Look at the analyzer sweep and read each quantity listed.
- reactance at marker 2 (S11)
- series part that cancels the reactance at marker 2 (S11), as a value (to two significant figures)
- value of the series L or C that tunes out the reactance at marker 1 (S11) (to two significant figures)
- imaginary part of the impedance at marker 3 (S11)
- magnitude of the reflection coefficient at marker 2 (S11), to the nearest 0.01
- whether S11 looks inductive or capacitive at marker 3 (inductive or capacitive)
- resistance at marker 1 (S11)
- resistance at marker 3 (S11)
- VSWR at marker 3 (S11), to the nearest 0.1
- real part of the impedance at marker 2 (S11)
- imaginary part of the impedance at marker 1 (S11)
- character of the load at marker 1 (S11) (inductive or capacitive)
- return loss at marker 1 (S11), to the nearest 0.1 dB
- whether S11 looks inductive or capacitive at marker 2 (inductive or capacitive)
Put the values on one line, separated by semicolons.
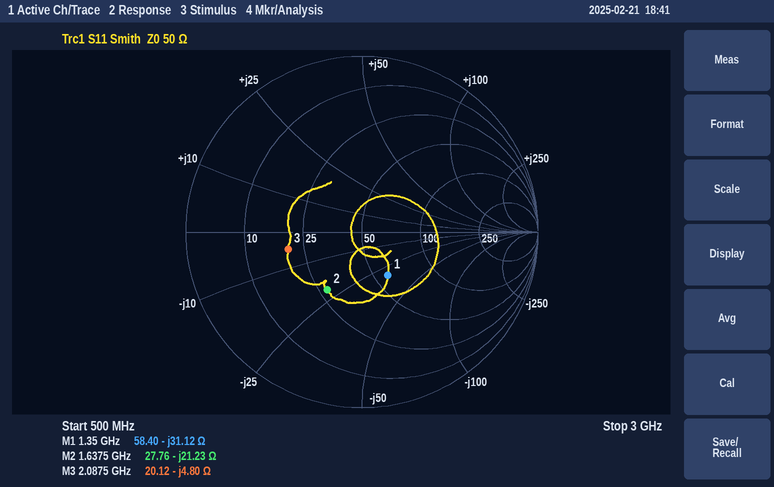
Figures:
-21.23 Ω; 2.1 nH; 3.7 nH; -4.80 Ω; 0.38; capacitive; 58.40 Ω; 20.12 Ω; 2.5; 27.76 Ω; -31.12 Ω; capacitive; 10.9 dB; capacitive
